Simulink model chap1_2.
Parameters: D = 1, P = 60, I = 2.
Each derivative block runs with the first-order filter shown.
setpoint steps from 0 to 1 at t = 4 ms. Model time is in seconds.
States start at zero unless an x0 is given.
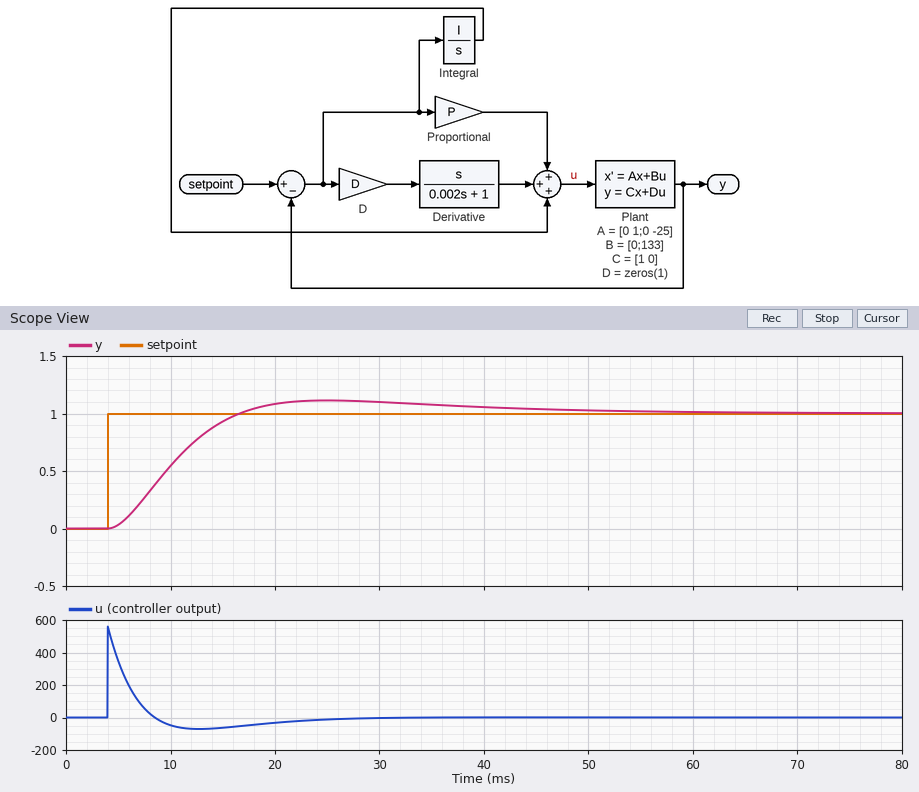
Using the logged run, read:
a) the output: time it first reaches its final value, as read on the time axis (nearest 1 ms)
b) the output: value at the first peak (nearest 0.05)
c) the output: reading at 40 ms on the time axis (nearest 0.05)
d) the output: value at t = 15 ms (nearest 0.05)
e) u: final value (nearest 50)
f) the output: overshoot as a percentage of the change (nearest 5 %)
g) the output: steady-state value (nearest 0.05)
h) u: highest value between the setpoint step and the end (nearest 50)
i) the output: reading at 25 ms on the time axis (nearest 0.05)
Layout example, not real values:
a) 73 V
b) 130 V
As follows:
a) 17 ms
b) 1.10
c) 1.05
d) 0.95
e) 0
f) 10 %
g) 1.00
h) 550
i) 1.10
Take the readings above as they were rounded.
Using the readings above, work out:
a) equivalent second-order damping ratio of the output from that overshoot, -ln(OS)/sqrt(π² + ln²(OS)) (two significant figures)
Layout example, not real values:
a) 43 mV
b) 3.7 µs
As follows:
a) 0.59
